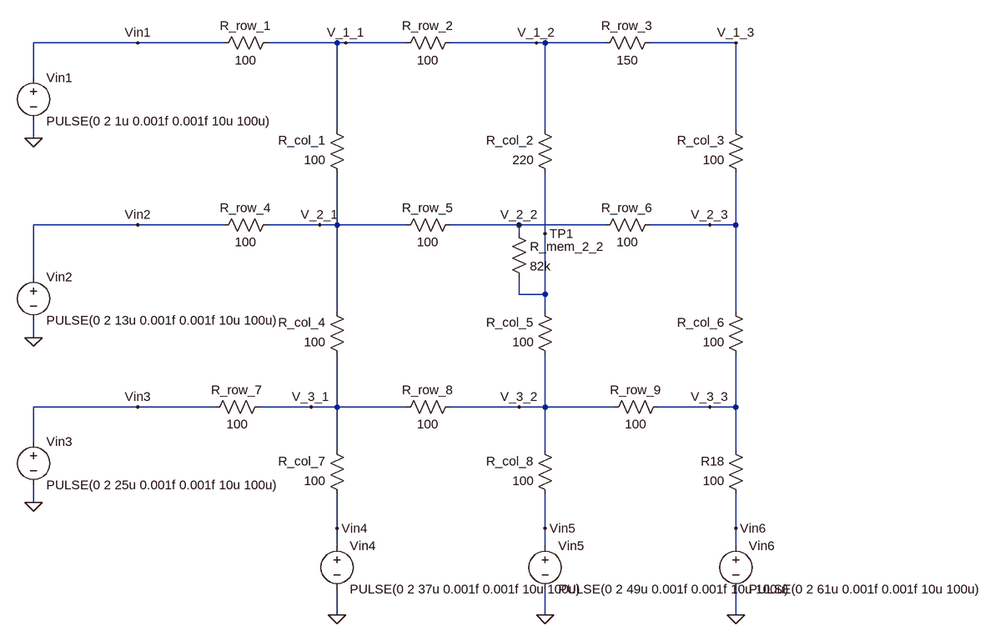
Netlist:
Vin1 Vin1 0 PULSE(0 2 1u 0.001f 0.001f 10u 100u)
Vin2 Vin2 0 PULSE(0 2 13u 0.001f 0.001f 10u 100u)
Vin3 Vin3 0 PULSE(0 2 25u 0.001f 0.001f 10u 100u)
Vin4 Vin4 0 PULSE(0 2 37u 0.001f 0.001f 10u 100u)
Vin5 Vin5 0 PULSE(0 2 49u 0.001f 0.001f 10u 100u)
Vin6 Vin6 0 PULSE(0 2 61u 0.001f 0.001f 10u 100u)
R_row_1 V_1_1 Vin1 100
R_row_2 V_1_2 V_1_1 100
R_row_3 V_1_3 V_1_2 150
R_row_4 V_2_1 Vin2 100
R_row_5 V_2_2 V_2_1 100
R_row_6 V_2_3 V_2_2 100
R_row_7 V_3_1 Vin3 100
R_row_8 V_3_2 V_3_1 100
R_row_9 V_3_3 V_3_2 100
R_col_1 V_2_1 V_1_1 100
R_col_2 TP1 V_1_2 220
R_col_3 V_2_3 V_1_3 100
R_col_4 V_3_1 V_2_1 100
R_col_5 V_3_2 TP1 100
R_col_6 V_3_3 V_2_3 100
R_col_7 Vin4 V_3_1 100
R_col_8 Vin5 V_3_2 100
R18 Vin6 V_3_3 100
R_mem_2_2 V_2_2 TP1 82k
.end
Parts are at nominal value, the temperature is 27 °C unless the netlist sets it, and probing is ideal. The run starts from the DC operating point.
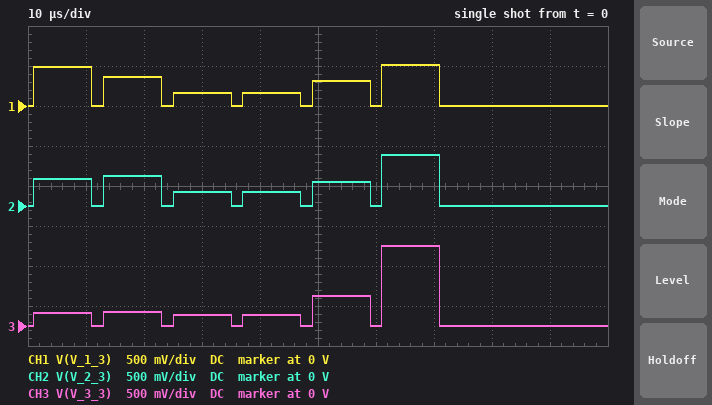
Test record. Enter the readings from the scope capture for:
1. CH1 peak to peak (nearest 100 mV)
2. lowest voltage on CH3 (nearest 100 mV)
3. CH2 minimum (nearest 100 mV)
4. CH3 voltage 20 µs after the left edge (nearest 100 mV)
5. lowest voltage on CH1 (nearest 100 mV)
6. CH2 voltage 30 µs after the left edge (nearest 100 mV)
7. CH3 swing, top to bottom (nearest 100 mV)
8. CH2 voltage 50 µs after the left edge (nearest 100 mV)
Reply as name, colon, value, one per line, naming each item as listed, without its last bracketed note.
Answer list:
CH1 peak to peak: 500 mV
lowest voltage on CH3: 0 V
CH2 minimum: 0 V
CH3 voltage 20 µs after the left edge: 200 mV
lowest voltage on CH1: 0 V
CH2 voltage 30 µs after the left edge: 200 mV
CH3 swing, top to bottom: 1.0 V
CH2 voltage 50 µs after the left edge: 300 mV
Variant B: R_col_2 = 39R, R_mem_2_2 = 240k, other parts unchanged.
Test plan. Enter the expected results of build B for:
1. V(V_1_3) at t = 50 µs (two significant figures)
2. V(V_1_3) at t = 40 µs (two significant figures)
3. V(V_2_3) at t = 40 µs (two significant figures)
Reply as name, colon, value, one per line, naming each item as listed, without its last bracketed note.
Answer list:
V(V_1_3) at t = 50 µs: 370 mV
V(V_1_3) at t = 40 µs: 180 mV
V(V_2_3) at t = 40 µs: 170 mV
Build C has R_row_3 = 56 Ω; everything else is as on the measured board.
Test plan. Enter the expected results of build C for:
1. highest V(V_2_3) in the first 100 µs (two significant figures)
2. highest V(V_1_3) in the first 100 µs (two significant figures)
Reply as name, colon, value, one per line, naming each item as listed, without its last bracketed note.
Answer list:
highest V(V_2_3) in the first 100 µs: 610 mV
highest V(V_1_3) in the first 100 µs: 560 mV
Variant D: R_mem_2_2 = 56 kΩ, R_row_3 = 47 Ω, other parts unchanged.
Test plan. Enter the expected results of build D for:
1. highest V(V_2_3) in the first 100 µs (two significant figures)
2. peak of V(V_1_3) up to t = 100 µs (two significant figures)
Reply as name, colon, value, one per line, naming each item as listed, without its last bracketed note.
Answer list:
highest V(V_2_3) in the first 100 µs: 610 mV
peak of V(V_1_3) up to t = 100 µs: 570 mV
